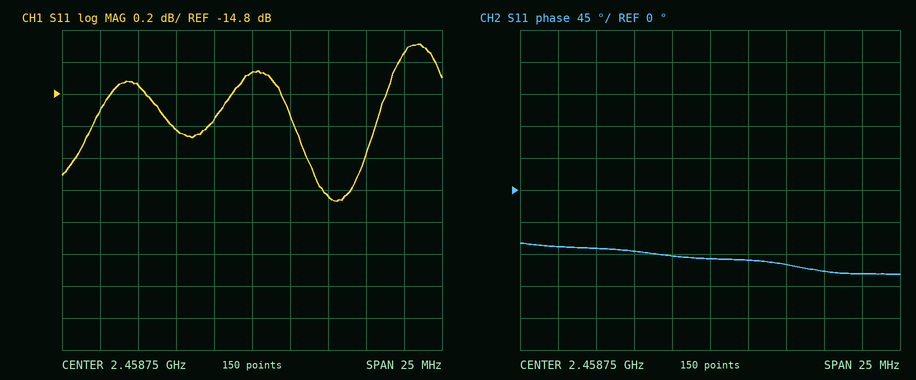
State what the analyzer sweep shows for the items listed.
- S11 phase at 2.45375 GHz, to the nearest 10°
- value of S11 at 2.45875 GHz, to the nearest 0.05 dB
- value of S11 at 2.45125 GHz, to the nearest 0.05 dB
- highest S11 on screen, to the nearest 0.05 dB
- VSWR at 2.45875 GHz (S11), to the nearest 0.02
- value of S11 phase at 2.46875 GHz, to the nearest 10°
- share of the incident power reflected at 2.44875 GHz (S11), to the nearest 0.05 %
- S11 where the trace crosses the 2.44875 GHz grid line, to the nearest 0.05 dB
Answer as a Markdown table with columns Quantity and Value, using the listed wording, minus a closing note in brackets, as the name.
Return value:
| Quantity | Value |
|---|---|
| S11 phase at 2.45375 GHz, to the nearest 10° | -90° |
| value of S11 at 2.45875 GHz, to the nearest 0.05 dB | -14.65 dB |
| value of S11 at 2.45125 GHz, to the nearest 0.05 dB | -14.75 dB |
| highest S11 on screen, to the nearest 0.05 dB | -14.50 dB |
| VSWR at 2.45875 GHz (S11), to the nearest 0.02 | 1.46 |
| value of S11 phase at 2.46875 GHz, to the nearest 10° | -120° |
| share of the incident power reflected at 2.44875 GHz (S11), to the nearest 0.05 % | 3.25 % |
| S11 where the trace crosses the 2.44875 GHz grid line, to the nearest 0.05 dB | -14.90 dB |
